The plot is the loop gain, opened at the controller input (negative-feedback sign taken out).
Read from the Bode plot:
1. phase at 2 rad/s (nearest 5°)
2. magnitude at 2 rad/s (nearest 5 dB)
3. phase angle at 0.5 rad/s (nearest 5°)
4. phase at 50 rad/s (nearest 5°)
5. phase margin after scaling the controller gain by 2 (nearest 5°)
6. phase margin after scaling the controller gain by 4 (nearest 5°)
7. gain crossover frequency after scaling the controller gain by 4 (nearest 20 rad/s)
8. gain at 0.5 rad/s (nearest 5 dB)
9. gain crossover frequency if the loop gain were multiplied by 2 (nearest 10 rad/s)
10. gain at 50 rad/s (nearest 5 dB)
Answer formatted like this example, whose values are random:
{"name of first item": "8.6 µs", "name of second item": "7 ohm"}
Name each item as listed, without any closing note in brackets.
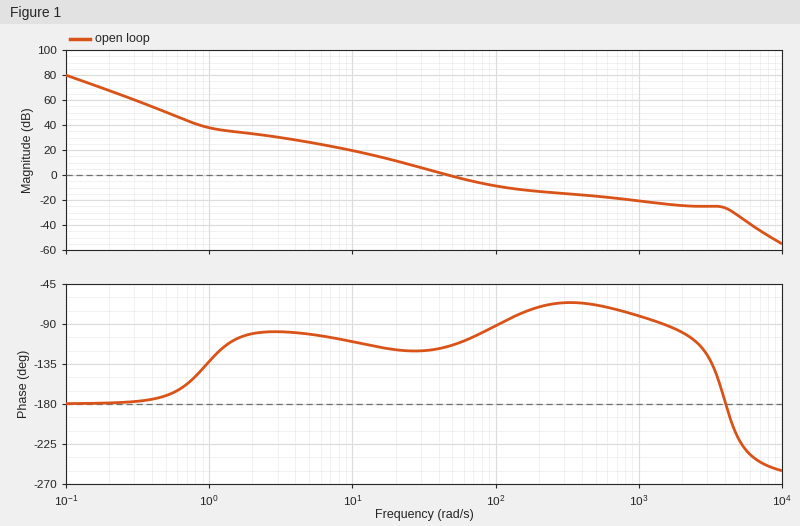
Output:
{"phase at 2 rad/s": "-100°", "magnitude at 2 rad/s": "35 dB", "phase angle at 0.5 rad/s": "-170°", "phase at 50 rad/s": "-115°", "phase margin after scaling the controller gain by 2": "80°", "phase margin after scaling the controller gain by 4": "105°", "gain crossover frequency after scaling the controller gain by 4": "160 rad/s", "gain at 0.5 rad/s": "50 dB", "gain crossover frequency if the loop gain were multiplied by 2": "80 rad/s", "gain at 50 rad/s": "0 dB"}
